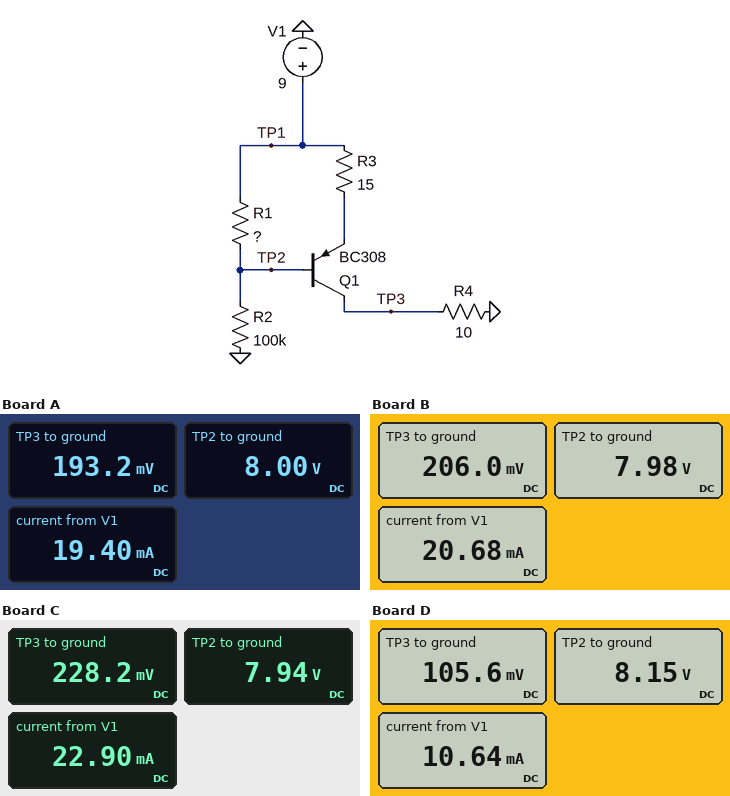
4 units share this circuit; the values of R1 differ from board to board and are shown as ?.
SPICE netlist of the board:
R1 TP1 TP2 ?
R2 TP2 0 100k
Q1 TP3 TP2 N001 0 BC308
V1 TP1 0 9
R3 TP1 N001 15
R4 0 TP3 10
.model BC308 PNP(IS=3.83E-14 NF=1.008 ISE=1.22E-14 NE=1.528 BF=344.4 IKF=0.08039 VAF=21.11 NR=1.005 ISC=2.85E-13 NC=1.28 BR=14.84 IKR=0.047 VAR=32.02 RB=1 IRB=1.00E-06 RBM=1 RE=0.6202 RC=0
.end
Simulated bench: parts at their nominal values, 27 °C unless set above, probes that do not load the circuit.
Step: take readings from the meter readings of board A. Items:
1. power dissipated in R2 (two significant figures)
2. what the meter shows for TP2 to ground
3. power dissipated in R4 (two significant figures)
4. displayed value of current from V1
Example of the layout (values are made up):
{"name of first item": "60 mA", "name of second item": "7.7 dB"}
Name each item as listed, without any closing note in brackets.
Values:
{"power dissipated in R2": "640 µW", "what the meter shows for TP2 to ground": "8.00 V", "power dissipated in R4": "3.7 mW", "displayed value of current from V1": "19.40 mA"}
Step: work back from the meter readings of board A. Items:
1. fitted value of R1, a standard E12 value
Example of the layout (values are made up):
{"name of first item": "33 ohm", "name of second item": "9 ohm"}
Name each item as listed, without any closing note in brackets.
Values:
{"fitted value of R1, a standard E12 value": "33 kΩ"}
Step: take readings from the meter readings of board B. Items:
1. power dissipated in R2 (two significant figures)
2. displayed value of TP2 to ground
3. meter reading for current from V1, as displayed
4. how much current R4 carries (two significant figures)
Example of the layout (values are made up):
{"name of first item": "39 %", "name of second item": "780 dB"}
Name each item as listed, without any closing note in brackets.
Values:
{"power dissipated in R2": "640 µW", "displayed value of TP2 to ground": "7.98 V", "meter reading for current from V1, as displayed": "20.68 mA", "how much current R4 carries": "21 mA"}
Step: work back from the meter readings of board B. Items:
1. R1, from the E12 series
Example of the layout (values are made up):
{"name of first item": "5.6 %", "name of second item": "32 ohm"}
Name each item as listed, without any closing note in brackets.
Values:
{"R1, from the E12 series": "39 kΩ"}
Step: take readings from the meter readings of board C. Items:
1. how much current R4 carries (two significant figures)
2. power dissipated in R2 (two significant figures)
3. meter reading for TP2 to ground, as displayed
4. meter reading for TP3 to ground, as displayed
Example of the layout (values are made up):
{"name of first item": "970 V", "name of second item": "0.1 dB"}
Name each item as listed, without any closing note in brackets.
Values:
{"how much current R4 carries": "23 mA", "power dissipated in R2": "630 µW", "meter reading for TP2 to ground, as displayed": "7.94 V", "meter reading for TP3 to ground, as displayed": "228.2 mV"}
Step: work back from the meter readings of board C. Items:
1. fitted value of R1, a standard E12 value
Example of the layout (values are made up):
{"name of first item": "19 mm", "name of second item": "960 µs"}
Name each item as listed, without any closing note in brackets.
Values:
{"fitted value of R1, a standard E12 value": "56 kΩ"}
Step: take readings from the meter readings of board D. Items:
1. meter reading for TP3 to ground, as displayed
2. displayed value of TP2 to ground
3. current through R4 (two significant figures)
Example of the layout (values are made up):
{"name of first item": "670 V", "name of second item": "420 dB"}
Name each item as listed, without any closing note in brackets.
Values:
{"meter reading for TP3 to ground, as displayed": "105.6 mV", "displayed value of TP2 to ground": "8.15 V", "current through R4": "11 mA"}
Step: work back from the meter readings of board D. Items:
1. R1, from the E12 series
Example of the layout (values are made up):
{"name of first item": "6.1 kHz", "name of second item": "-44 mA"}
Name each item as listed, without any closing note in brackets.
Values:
{"R1, from the E12 series": "15 kΩ"}
